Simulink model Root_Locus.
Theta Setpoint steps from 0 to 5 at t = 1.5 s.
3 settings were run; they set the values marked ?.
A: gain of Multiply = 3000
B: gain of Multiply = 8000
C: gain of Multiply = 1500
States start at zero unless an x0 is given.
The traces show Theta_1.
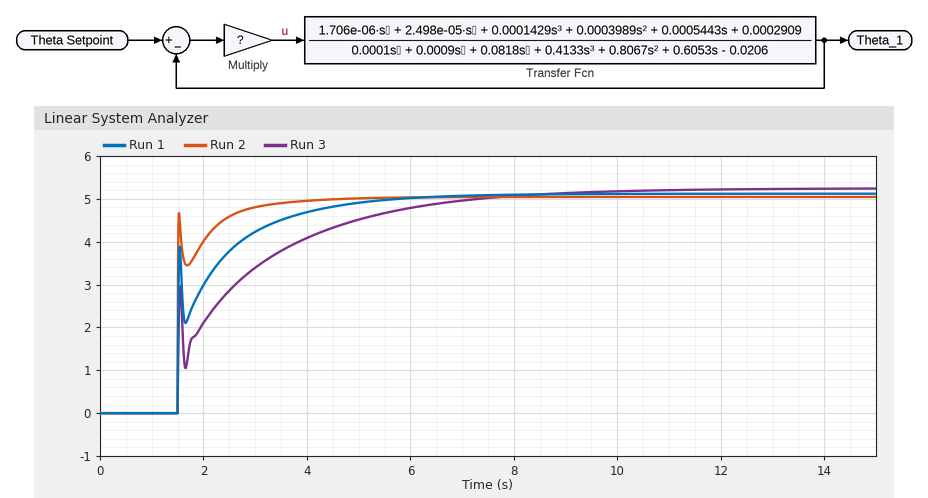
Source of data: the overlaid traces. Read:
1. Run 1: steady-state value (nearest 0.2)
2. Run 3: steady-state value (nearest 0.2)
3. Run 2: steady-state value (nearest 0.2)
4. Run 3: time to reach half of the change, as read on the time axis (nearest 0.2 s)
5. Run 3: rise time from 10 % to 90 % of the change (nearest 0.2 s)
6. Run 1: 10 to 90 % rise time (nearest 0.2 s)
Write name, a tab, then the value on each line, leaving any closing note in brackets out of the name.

Run 1: steady-state value	5.2
Run 3: steady-state value	5.2
Run 2: steady-state value	5.0
Run 3: time to reach half of the change, as read on the time axis	1.6 s
Run 3: rise time from 10 % to 90 % of the change	4.2 s
Run 1: 10 to 90 % rise time	2.2 s
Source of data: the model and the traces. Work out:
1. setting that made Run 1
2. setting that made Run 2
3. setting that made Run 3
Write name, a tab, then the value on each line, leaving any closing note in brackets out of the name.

setting that made Run 1	A
setting that made Run 2	B
setting that made Run 3	C
